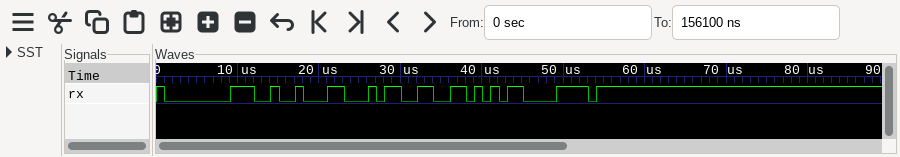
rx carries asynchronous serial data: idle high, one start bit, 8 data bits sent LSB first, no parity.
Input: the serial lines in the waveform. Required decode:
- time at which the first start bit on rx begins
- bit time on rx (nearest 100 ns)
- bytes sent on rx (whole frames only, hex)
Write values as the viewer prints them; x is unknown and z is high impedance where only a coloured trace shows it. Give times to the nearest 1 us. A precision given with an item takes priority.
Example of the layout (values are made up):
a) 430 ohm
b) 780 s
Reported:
a) 1 us
b) 1000 ns
c) 80, 12, 34, 56, 78
